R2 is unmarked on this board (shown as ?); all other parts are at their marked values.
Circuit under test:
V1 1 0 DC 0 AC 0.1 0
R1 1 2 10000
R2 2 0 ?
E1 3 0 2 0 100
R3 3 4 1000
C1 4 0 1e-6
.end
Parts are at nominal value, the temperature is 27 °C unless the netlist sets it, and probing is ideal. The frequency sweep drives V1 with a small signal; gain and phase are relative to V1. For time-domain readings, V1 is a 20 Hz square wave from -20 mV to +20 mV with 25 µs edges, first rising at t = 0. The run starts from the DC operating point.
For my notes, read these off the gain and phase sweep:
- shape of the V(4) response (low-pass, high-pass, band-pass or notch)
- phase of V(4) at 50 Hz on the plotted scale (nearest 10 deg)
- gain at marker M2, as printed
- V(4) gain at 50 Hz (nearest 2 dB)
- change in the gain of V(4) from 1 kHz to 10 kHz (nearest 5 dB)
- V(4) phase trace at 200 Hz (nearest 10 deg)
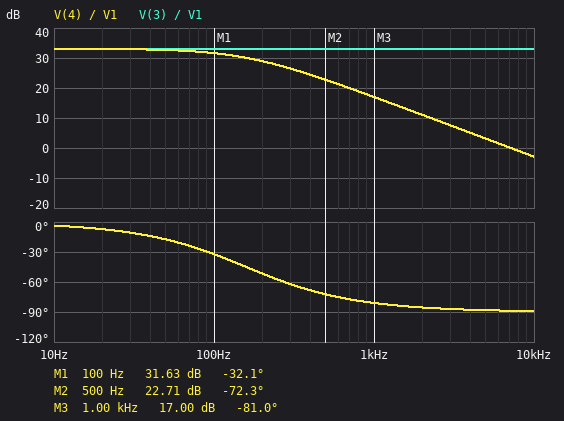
low-pass
-20 deg
22.71 dB
32 dB
-20 dB
-50 deg
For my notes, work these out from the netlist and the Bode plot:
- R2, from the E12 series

8.2 kΩ
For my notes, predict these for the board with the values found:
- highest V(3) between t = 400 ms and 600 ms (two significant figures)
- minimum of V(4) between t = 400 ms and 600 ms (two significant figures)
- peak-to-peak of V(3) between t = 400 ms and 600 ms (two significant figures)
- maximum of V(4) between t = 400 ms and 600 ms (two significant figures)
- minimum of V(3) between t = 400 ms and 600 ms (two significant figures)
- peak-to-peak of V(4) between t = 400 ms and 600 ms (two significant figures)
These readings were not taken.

900 mV
-900 mV
1.8 V
900 mV
-900 mV
1.8 V
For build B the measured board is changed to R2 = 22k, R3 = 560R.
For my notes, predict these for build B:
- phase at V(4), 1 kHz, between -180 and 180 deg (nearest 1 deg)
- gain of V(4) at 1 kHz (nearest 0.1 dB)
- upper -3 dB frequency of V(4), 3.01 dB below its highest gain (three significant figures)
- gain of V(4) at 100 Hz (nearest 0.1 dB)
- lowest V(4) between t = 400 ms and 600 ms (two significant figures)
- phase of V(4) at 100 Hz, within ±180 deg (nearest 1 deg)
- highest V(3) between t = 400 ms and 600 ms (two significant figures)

-74 deg
25.5 dB
284 Hz
36.2 dB
-1.4 V
-19 deg
1.4 V
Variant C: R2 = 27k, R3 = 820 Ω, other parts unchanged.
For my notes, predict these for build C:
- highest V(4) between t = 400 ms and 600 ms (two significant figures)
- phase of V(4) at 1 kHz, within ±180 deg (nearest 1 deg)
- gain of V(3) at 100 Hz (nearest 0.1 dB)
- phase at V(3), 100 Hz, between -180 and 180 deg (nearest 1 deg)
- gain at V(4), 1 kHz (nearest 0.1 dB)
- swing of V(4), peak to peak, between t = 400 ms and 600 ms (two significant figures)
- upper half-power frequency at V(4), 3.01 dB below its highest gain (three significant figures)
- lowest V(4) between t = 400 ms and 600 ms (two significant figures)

1.5 V
-79 deg
37.3 dB
0 deg
22.9 dB
2.9 V
194 Hz
-1.5 V
